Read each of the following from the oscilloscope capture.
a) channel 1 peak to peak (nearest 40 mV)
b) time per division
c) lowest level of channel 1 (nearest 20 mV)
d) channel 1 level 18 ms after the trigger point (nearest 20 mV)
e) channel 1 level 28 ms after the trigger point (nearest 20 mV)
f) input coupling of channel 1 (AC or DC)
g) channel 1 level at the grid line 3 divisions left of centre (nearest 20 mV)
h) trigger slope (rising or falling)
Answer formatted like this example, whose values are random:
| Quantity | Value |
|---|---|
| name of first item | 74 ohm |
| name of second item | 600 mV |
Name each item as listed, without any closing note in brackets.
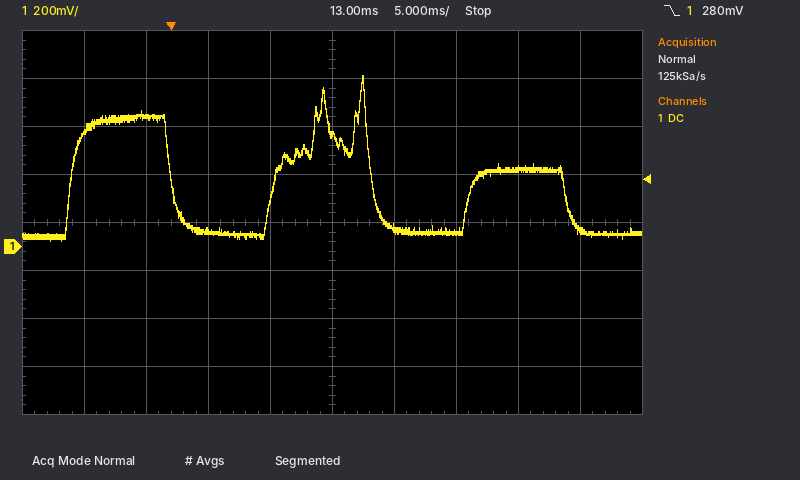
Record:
| Quantity | Value |
|---|---|
| channel 1 peak to peak | 680 mV |
| time per division | 5 ms |
| lowest level of channel 1 | 20 mV |
| channel 1 level 18 ms after the trigger point | 80 mV |
| channel 1 level 28 ms after the trigger point | 320 mV |
| input coupling of channel 1 | DC |
| channel 1 level at the grid line 3 divisions left of centre | 540 mV |
| trigger slope | falling |
